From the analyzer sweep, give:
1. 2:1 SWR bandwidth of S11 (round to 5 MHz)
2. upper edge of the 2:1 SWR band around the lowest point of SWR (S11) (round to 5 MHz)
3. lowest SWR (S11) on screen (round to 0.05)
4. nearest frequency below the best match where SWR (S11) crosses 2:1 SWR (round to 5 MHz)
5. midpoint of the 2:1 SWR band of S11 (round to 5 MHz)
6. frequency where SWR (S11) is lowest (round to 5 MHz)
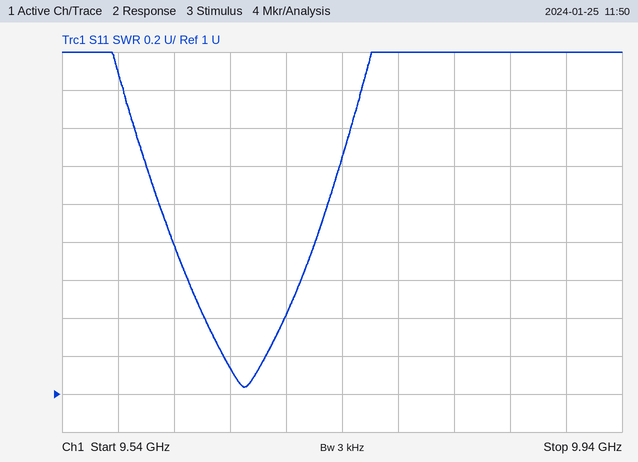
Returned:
120 MHz
9.730 GHz
1.05
9.610 GHz
9.670 GHz
9.670 GHz
